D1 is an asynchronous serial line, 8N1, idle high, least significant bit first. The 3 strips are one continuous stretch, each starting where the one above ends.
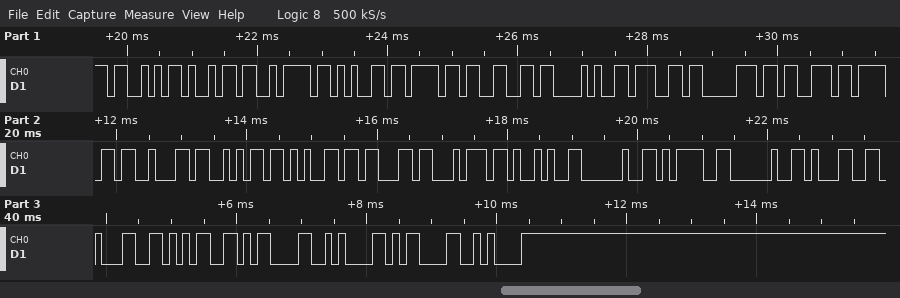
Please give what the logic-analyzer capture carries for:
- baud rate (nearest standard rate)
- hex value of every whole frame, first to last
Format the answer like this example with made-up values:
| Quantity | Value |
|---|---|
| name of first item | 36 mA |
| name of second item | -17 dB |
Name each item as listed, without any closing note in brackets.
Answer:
| Quantity | Value |
|---|---|
| baud rate | 9600 baud |
| hex value of every whole frame, first to last | 53 69 7A 65 6F 66 28 67 70 73 6F 62 6A 65 63 74 29 20 3D 20 31 31 35 0D 0A 0D 0A |
